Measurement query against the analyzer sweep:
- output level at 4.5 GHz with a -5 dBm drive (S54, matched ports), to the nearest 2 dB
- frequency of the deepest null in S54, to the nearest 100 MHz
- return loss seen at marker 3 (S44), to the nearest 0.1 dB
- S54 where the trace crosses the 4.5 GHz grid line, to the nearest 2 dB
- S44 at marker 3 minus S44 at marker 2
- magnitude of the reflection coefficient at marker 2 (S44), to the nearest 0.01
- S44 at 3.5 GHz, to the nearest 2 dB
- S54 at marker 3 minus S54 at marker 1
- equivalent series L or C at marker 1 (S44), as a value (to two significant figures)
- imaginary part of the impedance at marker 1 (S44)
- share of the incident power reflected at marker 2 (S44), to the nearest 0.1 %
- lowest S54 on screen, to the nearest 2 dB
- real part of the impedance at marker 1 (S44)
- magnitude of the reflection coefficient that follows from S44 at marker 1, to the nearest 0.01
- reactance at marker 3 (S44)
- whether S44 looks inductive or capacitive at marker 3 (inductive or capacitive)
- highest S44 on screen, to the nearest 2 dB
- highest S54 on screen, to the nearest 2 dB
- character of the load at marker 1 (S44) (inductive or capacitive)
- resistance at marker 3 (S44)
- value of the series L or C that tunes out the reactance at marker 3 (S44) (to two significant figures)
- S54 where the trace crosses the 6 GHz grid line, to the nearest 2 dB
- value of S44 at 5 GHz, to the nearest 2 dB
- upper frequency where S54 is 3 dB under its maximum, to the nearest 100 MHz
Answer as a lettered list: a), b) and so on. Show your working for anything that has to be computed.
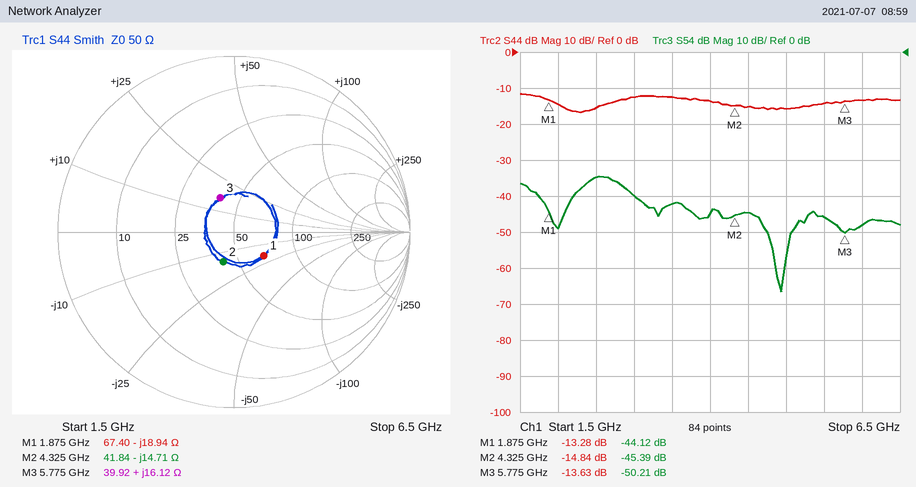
a) -5 dBm + (-44 dB) = -50 dBm
b) 4.9 GHz
c) 13.6 dB
d) -44 dB
e) -13.63 − (-14.84) = 1.21 dB
f) 0.18
g) -12 dB
h) -50.21 − (-44.12) = -6.09 dB
i) C = 1/(2π × 1.875 GHz × 18.94 Ω) ≈ 4.5 pF
j) -18.94 Ω
k) 10^(-14.84/10) ≈ 3.3 %
l) -66 dB
m) 67.40 Ω
n) 10^(-13.28/20) ≈ 0.22
o) +16.12 Ω
p) inductive
q) -12 dB
r) -34 dB
s) capacitive
t) 39.92 Ω
u) C = 1/(2π × 5.775 GHz × 16.12 Ω) ≈ 1.7 pF
v) -48 dB
w) -16 dB
x) 2.9 GHz
